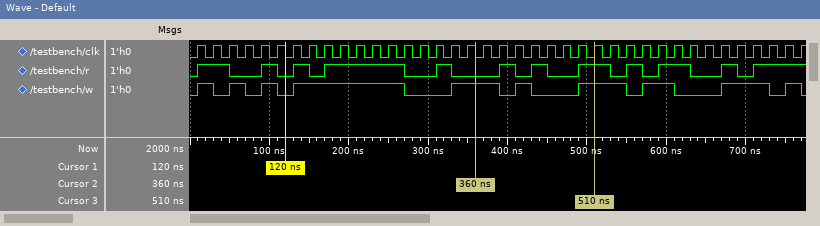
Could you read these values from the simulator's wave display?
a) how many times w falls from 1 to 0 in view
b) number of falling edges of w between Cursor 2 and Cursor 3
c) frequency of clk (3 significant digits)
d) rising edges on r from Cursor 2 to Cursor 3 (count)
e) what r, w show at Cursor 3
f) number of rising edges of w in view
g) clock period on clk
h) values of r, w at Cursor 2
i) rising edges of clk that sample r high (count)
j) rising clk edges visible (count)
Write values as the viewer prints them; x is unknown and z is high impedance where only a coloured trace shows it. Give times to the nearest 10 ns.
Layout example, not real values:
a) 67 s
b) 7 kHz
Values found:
a) 10
b) 2
c) 50.0 MHz
d) 3
e) r=1, w=1
f) 10
g) 20 ns
h) r=0, w=1
i) 21
j) 39
